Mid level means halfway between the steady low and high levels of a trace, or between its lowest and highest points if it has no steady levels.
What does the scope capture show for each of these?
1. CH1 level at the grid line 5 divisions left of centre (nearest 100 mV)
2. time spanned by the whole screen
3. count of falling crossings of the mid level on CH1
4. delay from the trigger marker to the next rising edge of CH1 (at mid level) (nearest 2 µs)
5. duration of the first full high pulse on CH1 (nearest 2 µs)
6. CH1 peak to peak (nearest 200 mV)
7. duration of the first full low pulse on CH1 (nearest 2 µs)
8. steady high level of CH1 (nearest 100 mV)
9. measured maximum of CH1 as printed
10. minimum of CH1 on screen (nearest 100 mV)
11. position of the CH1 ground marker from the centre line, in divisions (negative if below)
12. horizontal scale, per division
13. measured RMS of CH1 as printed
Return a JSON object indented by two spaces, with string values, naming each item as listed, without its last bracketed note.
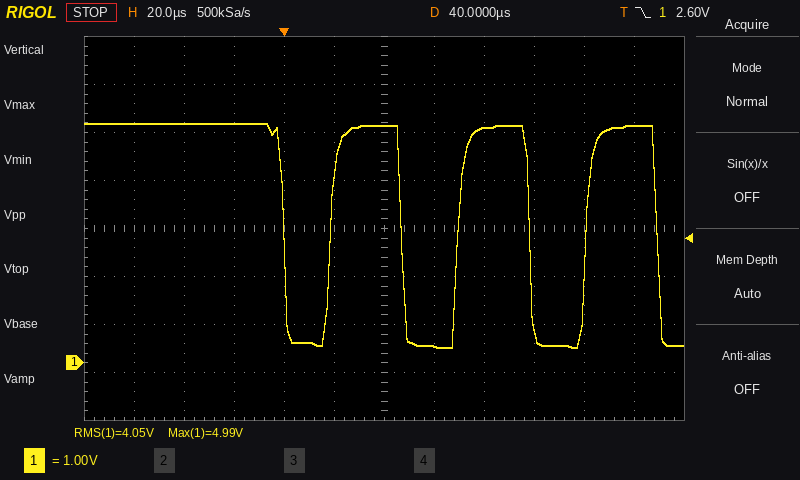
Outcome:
{
  "CH1 level at the grid line 5 divisions left of centre": "5.0 V",
  "time spanned by the whole screen": "240 µs",
  "count of falling crossings of the mid level on CH1": "4",
  "delay from the trigger marker to the next rising edge of CH1 (at mid level)": "18 µs",
  "duration of the first full high pulse on CH1": "28 µs",
  "CH1 peak to peak": "4.6 V",
  "duration of the first full low pulse on CH1": "18 µs",
  "steady high level of CH1": "5.0 V",
  "measured maximum of CH1 as printed": "4.99 V",
  "minimum of CH1 on screen": "300 mV",
  "position of the CH1 ground marker from the centre line, in divisions": "-2.8 div",
  "horizontal scale, per division": "20 µs",
  "measured RMS of CH1 as printed": "4.05 V"
}
